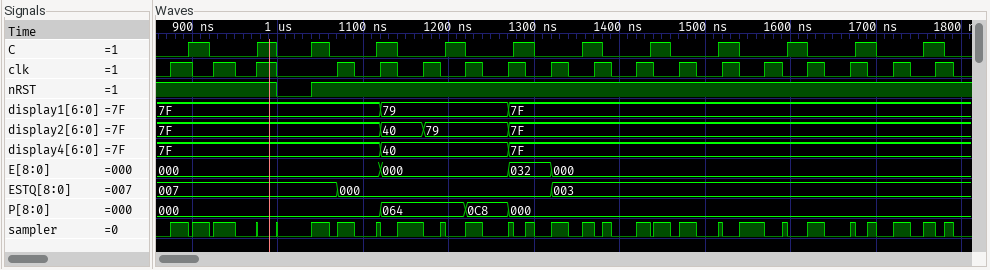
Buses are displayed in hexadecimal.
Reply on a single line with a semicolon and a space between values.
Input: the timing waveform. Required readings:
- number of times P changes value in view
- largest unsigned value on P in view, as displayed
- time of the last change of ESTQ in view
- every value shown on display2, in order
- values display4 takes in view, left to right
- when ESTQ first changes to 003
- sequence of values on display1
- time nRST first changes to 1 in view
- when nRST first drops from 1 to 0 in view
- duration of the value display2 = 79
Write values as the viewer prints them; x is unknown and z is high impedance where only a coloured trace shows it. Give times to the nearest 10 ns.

3; 0C8; 1320 ns; 7F, 40, 79, 7F; 7F, 40, 7F; 1320 ns; 7F, 79, 7F; 1040 ns; 1000 ns; 100 ns
